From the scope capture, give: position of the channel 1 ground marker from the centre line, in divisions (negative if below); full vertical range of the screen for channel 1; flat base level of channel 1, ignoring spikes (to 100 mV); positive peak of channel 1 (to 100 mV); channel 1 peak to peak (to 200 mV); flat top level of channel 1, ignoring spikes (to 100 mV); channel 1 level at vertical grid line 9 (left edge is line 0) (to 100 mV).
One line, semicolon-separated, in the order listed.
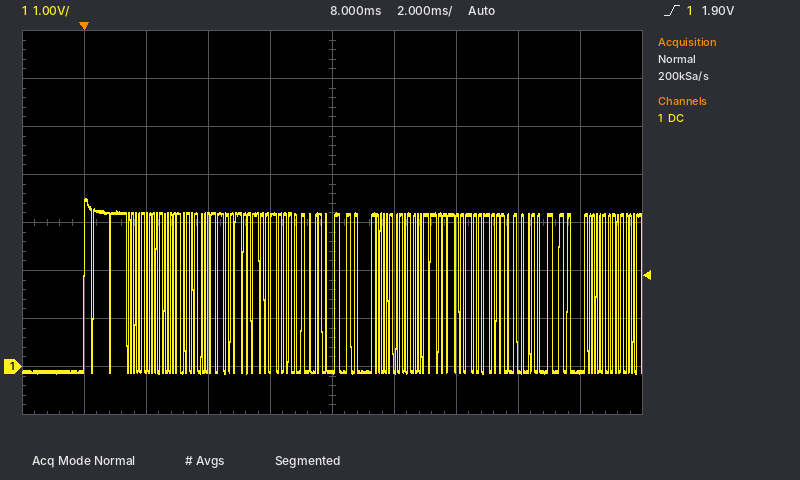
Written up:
-3.0 div; 8 V; -100 mV; 3.5 V; 3.6 V; 3.2 V; -100 mV
